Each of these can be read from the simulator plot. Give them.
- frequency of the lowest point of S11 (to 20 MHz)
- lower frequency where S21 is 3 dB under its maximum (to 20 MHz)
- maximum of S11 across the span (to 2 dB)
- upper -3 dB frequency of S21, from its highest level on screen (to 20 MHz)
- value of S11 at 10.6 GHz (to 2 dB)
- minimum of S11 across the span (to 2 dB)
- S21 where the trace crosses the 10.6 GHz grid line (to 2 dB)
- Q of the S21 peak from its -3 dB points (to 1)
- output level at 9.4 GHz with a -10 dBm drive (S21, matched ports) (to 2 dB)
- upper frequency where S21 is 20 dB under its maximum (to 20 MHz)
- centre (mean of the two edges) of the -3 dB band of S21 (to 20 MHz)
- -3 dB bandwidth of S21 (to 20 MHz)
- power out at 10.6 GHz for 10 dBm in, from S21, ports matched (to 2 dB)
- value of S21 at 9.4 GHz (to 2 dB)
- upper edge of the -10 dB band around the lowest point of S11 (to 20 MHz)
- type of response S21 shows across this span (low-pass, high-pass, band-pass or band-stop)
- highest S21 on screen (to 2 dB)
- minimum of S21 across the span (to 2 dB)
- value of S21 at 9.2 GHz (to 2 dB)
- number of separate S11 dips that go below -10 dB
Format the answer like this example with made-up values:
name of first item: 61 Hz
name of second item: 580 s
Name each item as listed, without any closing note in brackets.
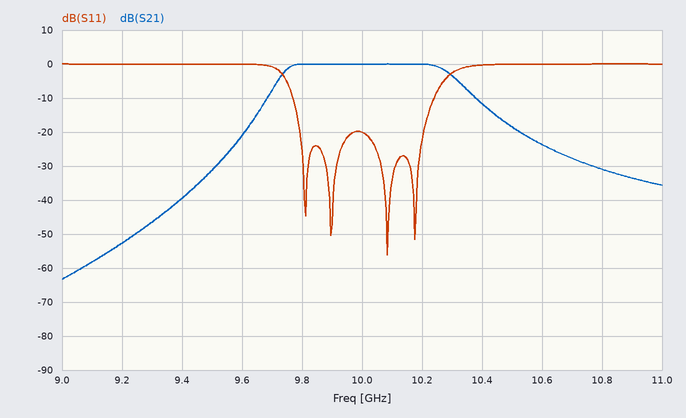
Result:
frequency of the lowest point of S11: 10.08 GHz
lower frequency where S21 is 3 dB under its maximum: 9.74 GHz
maximum of S11 across the span: 0 dB
upper -3 dB frequency of S21, from its highest level on screen: 10.30 GHz
value of S11 at 10.6 GHz: 0 dB
minimum of S11 across the span: -56 dB
S21 where the trace crosses the 10.6 GHz grid line: -24 dB
Q of the S21 peak from its -3 dB points: 18
output level at 9.4 GHz with a -10 dBm drive (S21, matched ports): -50 dBm
upper frequency where S21 is 20 dB under its maximum: 10.52 GHz
centre (mean of the two edges) of the -3 dB band of S21: 10.02 GHz
-3 dB bandwidth of S21: 560 MHz
power out at 10.6 GHz for 10 dBm in, from S21, ports matched: -14 dBm
value of S21 at 9.4 GHz: -40 dB
upper edge of the -10 dB band around the lowest point of S11: 10.24 GHz
type of response S21 shows across this span: band-pass
highest S21 on screen: 0 dB
minimum of S21 across the span: -64 dB
value of S21 at 9.2 GHz: -52 dB
number of separate S11 dips that go below -10 dB: 4
